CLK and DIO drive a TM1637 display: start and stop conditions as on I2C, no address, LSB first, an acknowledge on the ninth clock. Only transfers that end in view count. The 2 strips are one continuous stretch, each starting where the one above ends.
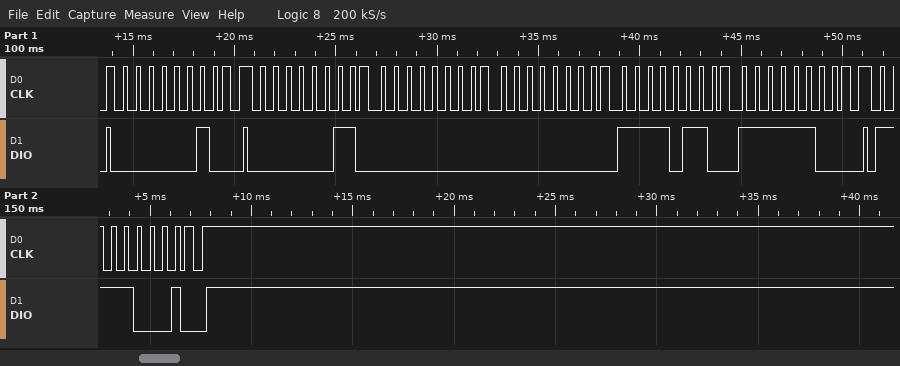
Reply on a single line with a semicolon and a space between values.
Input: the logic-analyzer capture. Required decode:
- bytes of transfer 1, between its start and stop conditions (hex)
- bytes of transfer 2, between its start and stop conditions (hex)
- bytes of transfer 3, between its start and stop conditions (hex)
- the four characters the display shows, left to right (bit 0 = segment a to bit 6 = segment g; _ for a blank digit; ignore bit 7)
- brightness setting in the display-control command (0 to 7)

40; C0 00 00 6F 3F; 8F; __90; 7
